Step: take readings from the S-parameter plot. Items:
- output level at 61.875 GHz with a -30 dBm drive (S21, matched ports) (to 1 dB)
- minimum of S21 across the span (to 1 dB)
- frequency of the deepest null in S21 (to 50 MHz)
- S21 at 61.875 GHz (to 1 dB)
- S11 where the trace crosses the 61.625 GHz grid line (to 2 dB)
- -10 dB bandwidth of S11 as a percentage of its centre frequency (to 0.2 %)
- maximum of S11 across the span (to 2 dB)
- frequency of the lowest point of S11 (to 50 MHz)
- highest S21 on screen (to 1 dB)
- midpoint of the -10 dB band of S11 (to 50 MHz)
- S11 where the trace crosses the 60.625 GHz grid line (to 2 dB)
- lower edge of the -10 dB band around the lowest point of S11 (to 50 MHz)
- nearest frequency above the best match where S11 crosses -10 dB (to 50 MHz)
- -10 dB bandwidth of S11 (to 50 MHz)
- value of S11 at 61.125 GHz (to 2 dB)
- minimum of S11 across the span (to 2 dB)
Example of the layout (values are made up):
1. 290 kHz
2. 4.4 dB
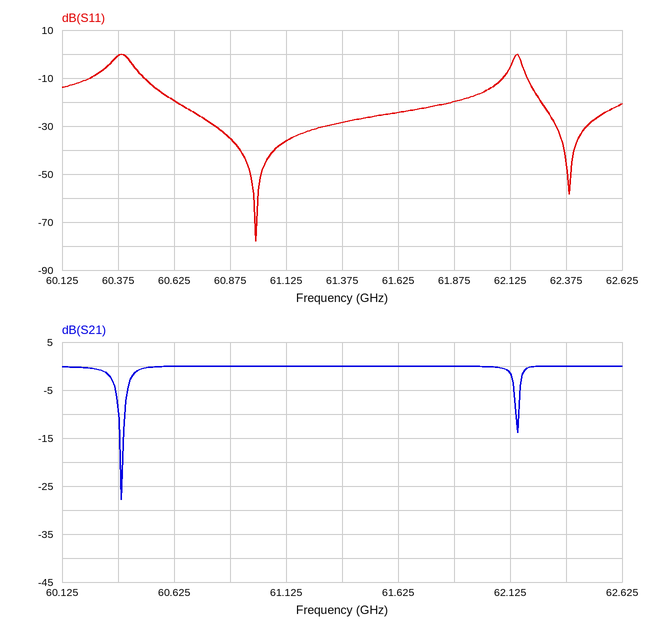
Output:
1. -30 dBm
2. -28 dB
3. 60.40 GHz
4. 0 dB
5. -24 dB
6. 2.6 %
7. 0 dB
8. 61.00 GHz
9. 0 dB
10. 61.30 GHz
11. -20 dB
12. 60.50 GHz
13. 62.10 GHz
14. 1.60 GHz
15. -36 dB
16. -78 dB
